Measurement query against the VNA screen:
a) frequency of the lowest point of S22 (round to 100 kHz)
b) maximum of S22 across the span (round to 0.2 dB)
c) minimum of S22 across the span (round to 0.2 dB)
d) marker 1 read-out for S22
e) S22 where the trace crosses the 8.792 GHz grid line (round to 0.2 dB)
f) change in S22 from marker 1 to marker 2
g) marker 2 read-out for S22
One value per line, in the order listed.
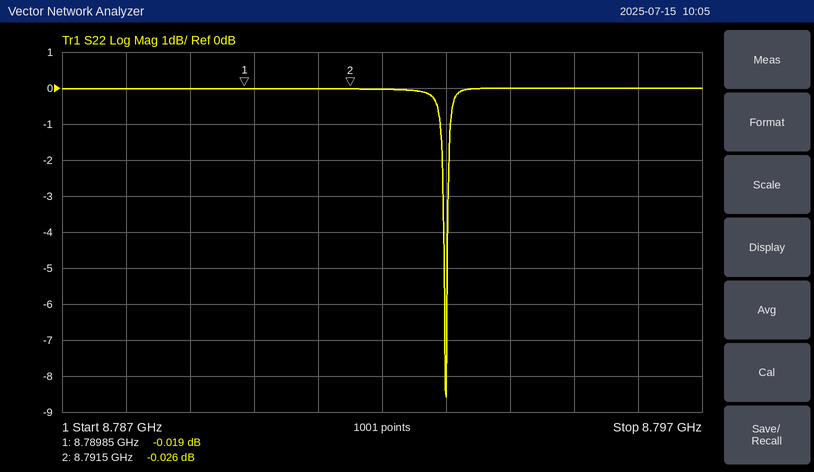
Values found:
8.7930 GHz
0.0 dB
-8.6 dB
-0.019 dB
0.0 dB
-0.007 dB
-0.026 dB
